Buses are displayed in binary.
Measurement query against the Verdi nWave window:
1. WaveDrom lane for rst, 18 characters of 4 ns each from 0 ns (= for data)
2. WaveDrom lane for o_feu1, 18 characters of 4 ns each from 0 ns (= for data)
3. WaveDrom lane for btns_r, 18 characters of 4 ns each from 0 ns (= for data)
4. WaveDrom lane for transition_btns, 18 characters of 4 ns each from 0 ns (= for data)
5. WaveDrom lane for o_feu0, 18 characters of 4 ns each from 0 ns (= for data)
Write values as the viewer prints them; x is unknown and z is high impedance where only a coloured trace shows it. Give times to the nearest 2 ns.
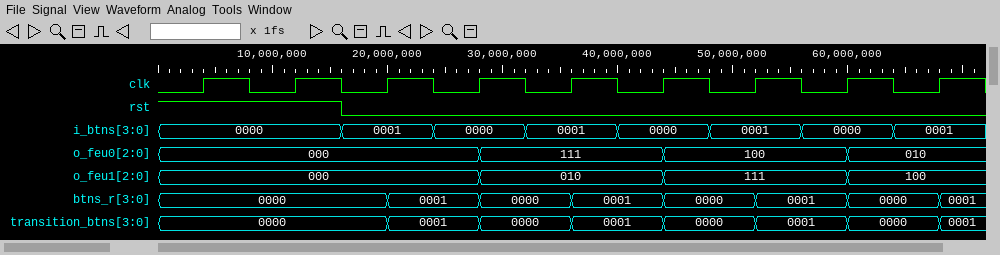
{name: 'rst', wave: '1...0.............'}
{name: 'o_feu1', wave: '=......=...=...=..', data: '000 010 111 100'}
{name: 'btns_r', wave: '=....=.=.=.=.=.=.=', data: '0000 0001 0000 0001 0000 0001 0000 0001'}
{name: 'transition_btns', wave: '=....=.=.=.=.=.=.=', data: '0000 0001 0000 0001 0000 0001 0000 0001'}
{name: 'o_feu0', wave: '=......=...=...=..', data: '000 111 100 010'}
